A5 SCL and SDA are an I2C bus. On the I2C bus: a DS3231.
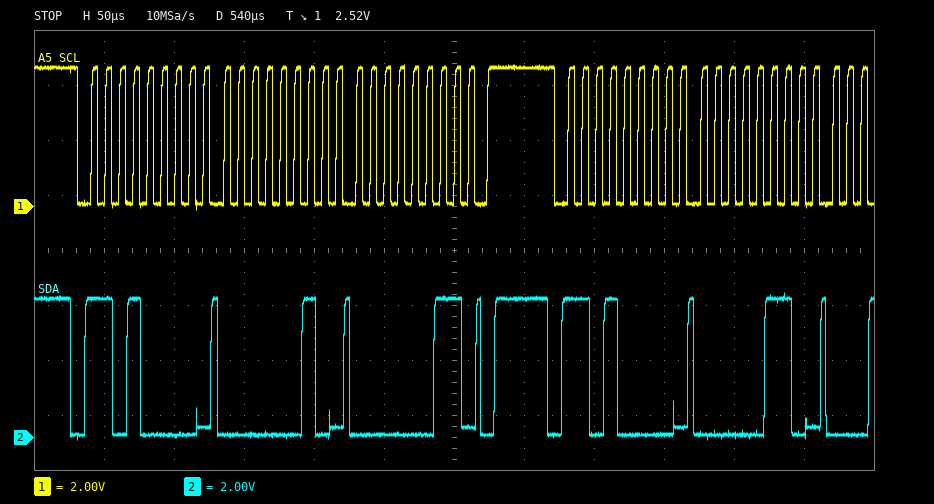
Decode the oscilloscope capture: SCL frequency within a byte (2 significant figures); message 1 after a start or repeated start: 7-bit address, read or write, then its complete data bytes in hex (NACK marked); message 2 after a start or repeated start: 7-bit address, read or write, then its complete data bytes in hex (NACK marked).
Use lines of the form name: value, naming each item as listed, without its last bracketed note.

SCL frequency within a byte: 100 kHz
message 1 after a start or repeated start: 7-bit address, read or write, then its complete data bytes in hex: 0x68 write: 02 03
message 2 after a start or repeated start: 7-bit address, read or write, then its complete data bytes in hex: 0x68 write: 06
